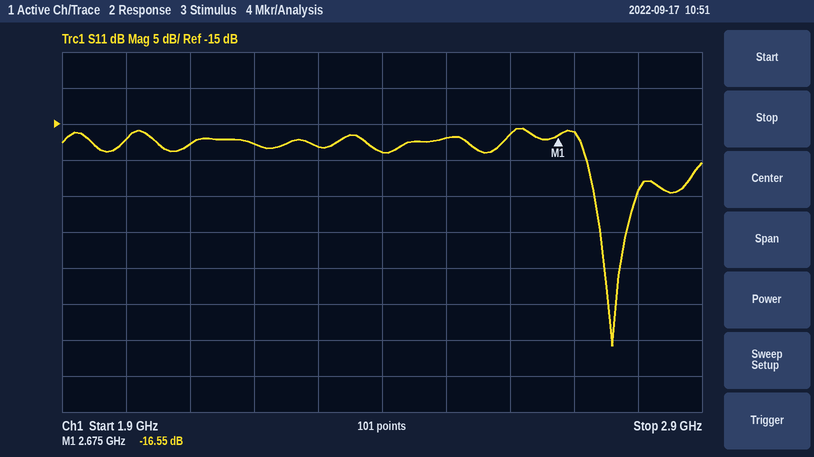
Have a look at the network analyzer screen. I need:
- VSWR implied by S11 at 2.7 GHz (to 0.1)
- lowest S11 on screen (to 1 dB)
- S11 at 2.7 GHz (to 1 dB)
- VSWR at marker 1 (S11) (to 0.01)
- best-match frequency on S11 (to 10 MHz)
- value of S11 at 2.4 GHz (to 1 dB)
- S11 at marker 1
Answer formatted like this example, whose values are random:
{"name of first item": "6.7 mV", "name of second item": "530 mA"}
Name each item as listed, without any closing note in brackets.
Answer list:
{"VSWR implied by S11 at 2.7 GHz": "1.4", "lowest S11 on screen": "-46 dB", "S11 at 2.7 GHz": "-16 dB", "VSWR at marker 1 (S11)": "1.35", "best-match frequency on S11": "2.76 GHz", "value of S11 at 2.4 GHz": "-19 dB", "S11 at marker 1": "-16.55 dB"}
